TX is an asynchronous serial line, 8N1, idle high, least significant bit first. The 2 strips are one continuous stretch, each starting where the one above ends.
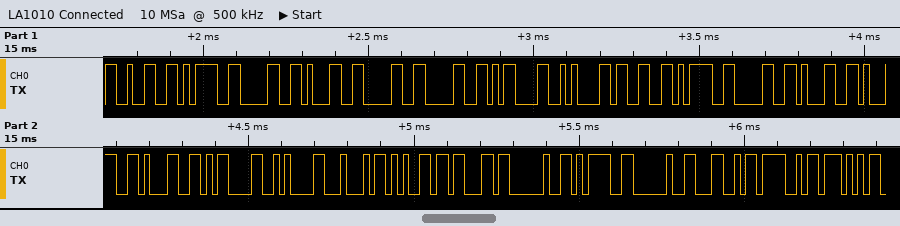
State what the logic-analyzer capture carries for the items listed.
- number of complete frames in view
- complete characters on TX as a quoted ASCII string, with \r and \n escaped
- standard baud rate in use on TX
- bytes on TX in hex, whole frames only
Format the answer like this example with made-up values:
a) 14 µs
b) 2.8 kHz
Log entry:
a) 25
b) "2=0100\r\n3=0111\r\nDec = LOW"
c) 57600 baud
d) 32 3D 30 31 30 30 0D 0A 33 3D 30 31 31 31 0D 0A 44 65 63 20 3D 20 4C 4F 57
